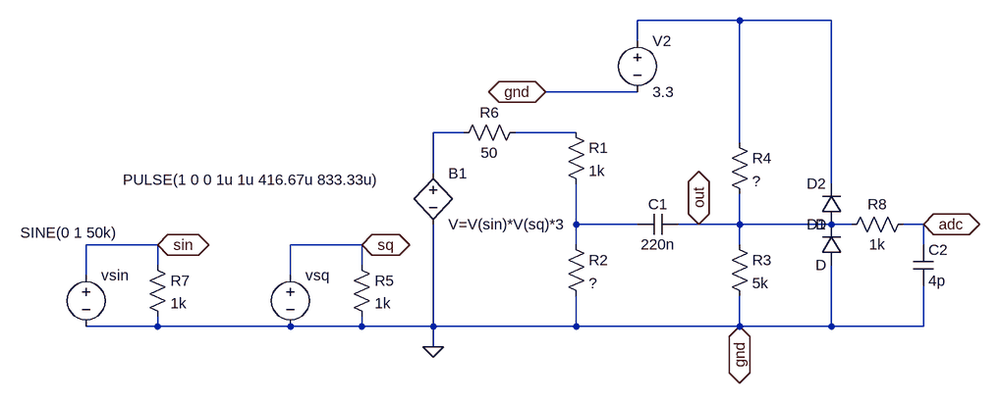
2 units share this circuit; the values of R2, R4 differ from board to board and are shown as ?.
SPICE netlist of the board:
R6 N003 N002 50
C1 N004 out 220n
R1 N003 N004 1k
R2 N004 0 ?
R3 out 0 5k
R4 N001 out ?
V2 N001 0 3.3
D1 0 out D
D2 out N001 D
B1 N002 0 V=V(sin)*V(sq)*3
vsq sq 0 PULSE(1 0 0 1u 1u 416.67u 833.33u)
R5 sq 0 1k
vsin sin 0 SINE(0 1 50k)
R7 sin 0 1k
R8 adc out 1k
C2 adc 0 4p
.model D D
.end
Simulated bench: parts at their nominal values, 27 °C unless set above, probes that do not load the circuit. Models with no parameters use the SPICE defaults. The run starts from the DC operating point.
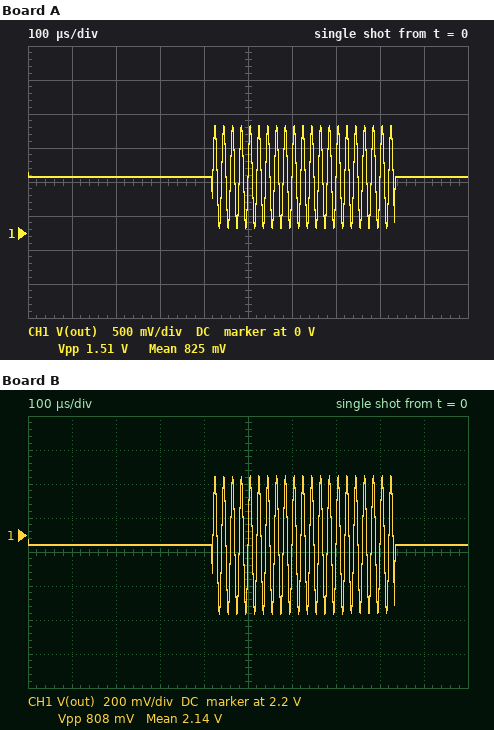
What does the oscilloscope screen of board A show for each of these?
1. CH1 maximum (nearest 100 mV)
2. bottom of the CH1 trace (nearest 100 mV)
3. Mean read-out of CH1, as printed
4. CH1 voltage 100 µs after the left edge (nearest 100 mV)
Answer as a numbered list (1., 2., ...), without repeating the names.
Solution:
1. 1.6 V
2. 100 mV
3. 825 mV
4. 800 mV
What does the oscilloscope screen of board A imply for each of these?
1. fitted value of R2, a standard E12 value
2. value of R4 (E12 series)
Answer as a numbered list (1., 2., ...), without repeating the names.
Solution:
1. 390 Ω
2. 15 kΩ
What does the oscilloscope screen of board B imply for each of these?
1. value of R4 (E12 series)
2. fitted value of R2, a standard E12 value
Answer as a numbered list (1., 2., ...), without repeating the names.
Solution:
1. 2.7 kΩ
2. 180 Ω
